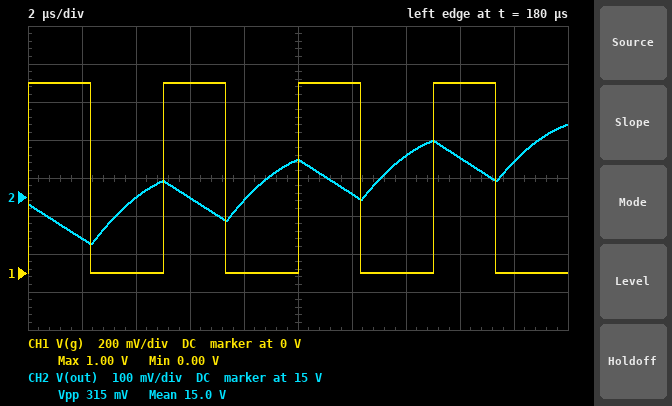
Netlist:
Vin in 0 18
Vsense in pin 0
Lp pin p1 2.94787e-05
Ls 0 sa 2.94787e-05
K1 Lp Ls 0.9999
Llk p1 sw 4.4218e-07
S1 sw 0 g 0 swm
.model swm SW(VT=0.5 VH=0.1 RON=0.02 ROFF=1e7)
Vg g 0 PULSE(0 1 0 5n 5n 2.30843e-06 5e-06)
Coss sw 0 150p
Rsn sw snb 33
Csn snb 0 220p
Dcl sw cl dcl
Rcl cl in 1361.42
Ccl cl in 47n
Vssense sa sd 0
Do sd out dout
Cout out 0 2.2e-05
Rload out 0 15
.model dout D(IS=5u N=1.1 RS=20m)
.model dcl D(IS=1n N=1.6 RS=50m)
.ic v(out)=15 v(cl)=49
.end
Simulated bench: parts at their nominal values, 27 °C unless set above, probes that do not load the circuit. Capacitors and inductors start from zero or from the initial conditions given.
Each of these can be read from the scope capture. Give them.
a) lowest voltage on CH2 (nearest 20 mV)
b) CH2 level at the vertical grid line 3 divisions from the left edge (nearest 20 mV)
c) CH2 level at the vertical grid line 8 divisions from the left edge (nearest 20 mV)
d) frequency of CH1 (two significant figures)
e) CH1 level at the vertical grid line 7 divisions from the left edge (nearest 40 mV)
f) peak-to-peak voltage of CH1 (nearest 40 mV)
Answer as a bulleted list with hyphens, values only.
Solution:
- 14.88 V
- 15.00 V
- 15.10 V
- 200 kHz
- 0 V
- 1.00 V
